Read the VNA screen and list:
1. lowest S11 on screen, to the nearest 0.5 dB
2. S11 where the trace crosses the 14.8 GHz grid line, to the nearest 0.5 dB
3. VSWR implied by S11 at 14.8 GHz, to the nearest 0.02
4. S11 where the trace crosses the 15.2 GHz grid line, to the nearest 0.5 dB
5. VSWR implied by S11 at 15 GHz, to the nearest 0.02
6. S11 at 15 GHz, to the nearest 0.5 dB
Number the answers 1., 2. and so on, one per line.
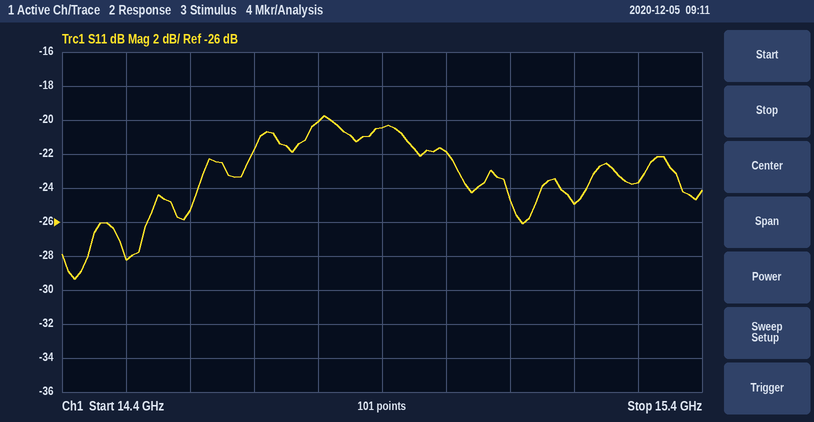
1. -29.5 dB
2. -20.0 dB
3. 1.22
4. -25.0 dB
5. 1.18
6. -22.0 dB
